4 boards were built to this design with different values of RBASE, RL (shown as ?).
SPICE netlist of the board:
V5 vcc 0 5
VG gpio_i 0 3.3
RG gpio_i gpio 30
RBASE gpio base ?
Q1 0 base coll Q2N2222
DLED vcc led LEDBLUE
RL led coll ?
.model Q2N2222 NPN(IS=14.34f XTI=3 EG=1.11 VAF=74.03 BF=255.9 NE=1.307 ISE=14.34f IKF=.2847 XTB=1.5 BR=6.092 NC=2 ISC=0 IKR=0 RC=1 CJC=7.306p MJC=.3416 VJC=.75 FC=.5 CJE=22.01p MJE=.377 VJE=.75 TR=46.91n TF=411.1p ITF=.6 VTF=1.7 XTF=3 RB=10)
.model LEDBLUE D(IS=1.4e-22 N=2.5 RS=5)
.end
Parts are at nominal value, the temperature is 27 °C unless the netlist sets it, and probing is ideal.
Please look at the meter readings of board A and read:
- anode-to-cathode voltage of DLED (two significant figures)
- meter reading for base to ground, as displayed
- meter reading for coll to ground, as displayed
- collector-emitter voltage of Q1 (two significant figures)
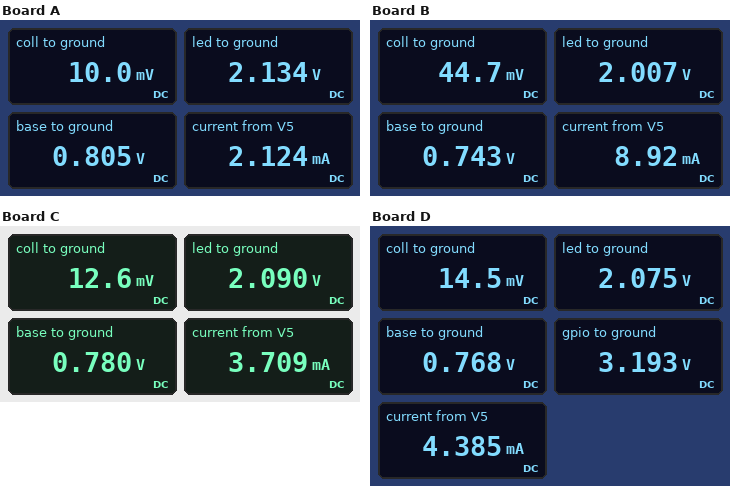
2.9 V
0.805 V
10.0 mV
-10 mV
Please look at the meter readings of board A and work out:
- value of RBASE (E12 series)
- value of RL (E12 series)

390 Ω
1 kΩ
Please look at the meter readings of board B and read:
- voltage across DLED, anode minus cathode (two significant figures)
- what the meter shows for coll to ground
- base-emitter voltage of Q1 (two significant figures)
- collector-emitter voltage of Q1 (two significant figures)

3.0 V
44.7 mV
700 mV
-45 mV
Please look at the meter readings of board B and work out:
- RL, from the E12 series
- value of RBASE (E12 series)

220 Ω
1.2 kΩ
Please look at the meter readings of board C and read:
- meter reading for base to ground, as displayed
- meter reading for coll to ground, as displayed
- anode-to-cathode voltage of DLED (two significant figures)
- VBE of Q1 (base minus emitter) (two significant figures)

0.780 V
12.6 mV
2.9 V
770 mV
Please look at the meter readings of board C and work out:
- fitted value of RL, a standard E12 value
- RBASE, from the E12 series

560 Ω
560 Ω
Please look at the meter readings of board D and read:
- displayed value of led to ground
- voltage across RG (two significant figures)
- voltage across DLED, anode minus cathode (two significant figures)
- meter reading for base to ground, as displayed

2.075 V
110 mV
2.9 V
0.768 V
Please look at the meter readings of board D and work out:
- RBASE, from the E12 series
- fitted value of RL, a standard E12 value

680 Ω
470 Ω
